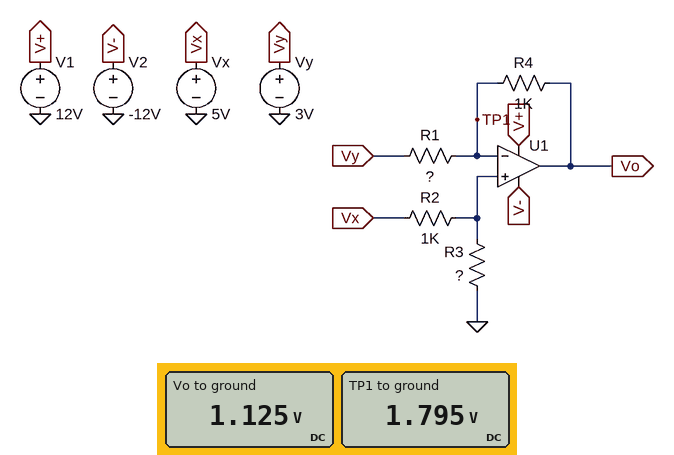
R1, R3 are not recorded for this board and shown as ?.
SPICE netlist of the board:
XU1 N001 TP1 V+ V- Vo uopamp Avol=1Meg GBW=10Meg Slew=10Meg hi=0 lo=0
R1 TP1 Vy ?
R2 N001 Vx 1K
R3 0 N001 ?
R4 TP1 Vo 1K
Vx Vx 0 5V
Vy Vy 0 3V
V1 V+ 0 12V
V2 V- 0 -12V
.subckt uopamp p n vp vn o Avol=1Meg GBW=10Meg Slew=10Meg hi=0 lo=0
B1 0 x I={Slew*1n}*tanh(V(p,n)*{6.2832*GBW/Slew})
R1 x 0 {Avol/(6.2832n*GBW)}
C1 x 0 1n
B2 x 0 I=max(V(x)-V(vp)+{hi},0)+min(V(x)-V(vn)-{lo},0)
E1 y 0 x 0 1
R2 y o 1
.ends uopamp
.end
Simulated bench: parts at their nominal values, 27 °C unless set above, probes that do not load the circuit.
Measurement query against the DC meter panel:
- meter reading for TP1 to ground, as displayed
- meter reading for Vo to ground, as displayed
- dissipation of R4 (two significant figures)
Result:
1.795 V
1.125 V
450 µW
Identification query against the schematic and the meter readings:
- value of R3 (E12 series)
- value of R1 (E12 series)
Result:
560 Ω
1.8 kΩ
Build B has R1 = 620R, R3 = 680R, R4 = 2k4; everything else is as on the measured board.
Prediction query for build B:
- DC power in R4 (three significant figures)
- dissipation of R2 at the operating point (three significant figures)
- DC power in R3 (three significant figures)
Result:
5.95 mW
8.86 mW
6.02 mW
